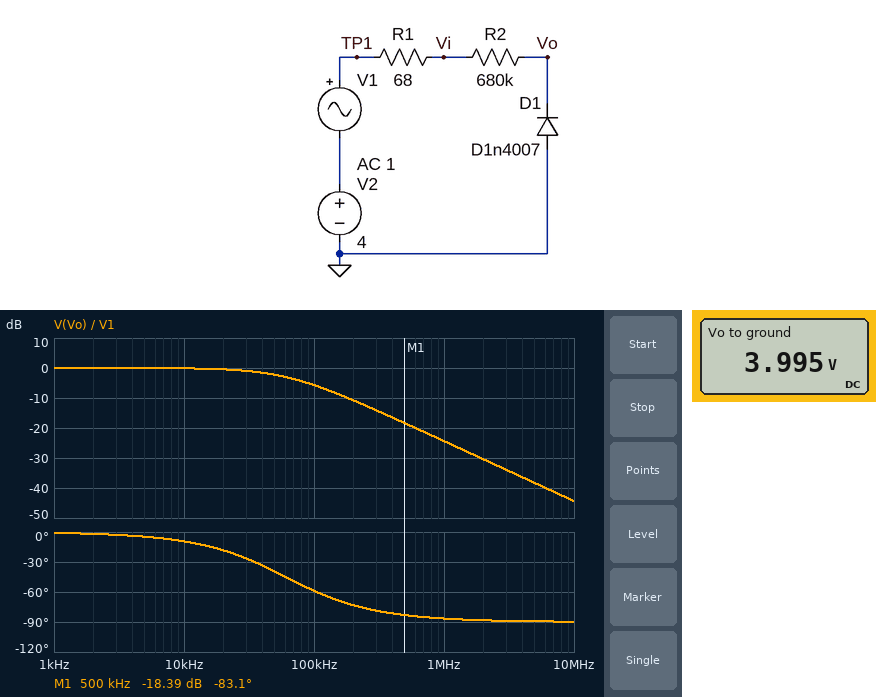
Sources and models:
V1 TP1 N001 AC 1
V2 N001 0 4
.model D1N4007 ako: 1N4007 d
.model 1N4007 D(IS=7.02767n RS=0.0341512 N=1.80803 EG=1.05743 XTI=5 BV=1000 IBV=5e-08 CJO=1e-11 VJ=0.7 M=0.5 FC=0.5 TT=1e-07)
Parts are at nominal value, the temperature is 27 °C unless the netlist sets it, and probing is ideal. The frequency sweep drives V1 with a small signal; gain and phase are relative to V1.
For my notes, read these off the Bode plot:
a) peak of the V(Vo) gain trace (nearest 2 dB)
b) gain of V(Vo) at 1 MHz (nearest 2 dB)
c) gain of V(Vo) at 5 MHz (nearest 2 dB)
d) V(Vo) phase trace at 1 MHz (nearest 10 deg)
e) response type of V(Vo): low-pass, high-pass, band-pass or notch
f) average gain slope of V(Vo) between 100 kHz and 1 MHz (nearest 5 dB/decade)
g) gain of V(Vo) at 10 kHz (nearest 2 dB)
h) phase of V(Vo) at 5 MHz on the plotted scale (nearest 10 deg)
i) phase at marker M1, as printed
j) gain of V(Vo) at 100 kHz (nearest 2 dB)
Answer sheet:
0 dB
-24 dB
-38 dB
-90 deg
low-pass
-20 dB/decade
0 dB
-90 deg
-83.1 deg
-6 dB
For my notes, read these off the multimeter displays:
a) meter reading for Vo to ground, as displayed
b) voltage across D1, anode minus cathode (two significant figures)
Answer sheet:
3.995 V
-4.0 V
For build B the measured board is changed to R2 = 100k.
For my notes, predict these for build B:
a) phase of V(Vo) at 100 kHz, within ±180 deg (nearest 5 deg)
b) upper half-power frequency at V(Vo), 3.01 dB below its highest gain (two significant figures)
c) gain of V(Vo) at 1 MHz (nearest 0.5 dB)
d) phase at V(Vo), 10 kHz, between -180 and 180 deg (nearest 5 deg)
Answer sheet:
-15 deg
410 kHz
-8.5 dB
0 deg
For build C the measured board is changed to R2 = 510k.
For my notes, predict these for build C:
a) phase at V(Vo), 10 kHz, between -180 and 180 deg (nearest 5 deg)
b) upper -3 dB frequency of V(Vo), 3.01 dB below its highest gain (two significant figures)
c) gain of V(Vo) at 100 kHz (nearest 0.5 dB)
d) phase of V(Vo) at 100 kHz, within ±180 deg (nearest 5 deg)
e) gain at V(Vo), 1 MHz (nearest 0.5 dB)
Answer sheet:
-5 deg
81 kHz
-4.0 dB
-50 deg
-22.0 dB
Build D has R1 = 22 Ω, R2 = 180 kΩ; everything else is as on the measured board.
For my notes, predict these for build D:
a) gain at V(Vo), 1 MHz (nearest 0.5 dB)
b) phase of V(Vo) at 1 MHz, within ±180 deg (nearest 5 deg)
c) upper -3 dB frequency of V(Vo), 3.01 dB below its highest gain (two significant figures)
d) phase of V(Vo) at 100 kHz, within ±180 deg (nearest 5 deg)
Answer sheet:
-13.0 dB
-75 deg
230 kHz
-25 deg
